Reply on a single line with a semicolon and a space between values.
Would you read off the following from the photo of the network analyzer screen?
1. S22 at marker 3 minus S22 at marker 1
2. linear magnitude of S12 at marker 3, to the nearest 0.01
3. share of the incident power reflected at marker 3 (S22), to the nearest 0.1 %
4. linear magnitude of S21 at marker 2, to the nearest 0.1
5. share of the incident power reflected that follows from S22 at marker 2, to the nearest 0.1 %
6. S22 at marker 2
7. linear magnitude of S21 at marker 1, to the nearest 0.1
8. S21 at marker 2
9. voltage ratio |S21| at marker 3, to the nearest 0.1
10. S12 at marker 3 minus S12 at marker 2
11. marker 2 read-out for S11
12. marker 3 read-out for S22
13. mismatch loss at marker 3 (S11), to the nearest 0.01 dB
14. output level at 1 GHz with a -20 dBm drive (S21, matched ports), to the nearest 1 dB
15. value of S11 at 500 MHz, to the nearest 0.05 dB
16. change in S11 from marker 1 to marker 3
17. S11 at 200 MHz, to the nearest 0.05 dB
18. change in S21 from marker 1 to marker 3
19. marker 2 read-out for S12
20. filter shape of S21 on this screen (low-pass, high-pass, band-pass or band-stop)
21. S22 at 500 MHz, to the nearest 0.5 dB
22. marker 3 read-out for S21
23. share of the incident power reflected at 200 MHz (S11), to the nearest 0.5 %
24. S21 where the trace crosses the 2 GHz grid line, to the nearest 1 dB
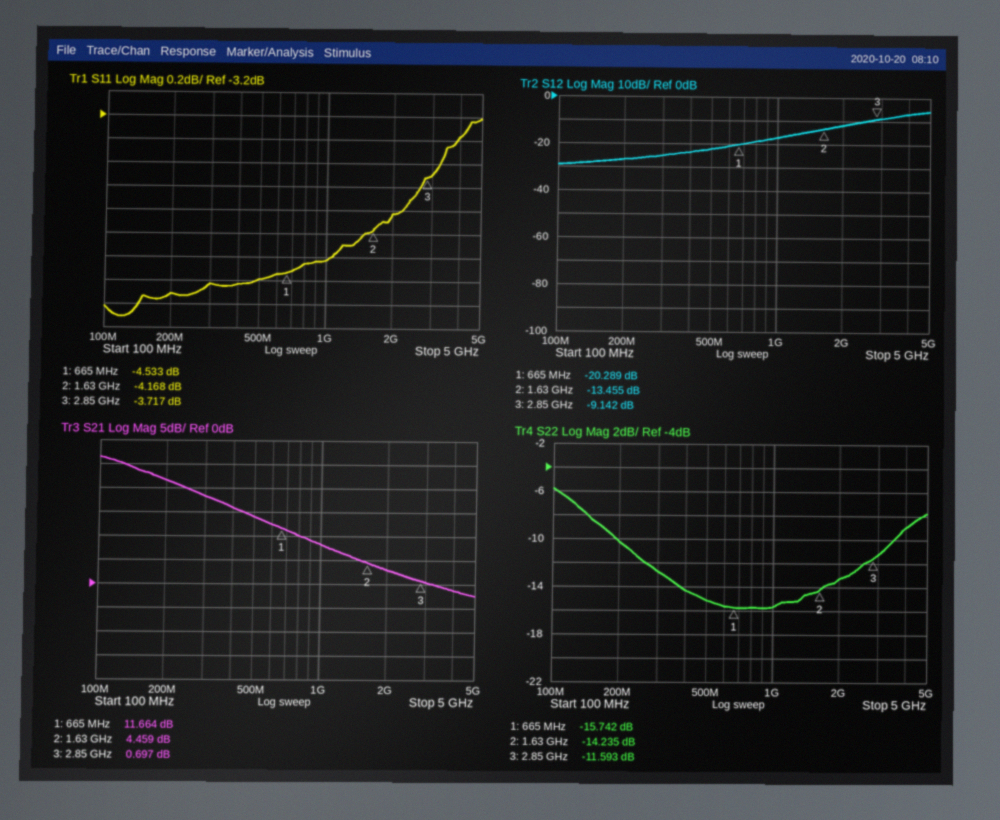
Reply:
4.149 dB; 0.35; 6.9 %; 1.7; 3.8 %; -14.235 dB; 3.8; 4.459 dB; 1.1; 4.313 dB; -4.168 dB; -11.593 dB; 2.40 dB; -12 dBm; -4.60 dB; 0.816 dB; -4.70 dB; -10.967 dB; -13.455 dB; low-pass; -15.0 dB; 0.697 dB; 34.0 %; 3 dB
